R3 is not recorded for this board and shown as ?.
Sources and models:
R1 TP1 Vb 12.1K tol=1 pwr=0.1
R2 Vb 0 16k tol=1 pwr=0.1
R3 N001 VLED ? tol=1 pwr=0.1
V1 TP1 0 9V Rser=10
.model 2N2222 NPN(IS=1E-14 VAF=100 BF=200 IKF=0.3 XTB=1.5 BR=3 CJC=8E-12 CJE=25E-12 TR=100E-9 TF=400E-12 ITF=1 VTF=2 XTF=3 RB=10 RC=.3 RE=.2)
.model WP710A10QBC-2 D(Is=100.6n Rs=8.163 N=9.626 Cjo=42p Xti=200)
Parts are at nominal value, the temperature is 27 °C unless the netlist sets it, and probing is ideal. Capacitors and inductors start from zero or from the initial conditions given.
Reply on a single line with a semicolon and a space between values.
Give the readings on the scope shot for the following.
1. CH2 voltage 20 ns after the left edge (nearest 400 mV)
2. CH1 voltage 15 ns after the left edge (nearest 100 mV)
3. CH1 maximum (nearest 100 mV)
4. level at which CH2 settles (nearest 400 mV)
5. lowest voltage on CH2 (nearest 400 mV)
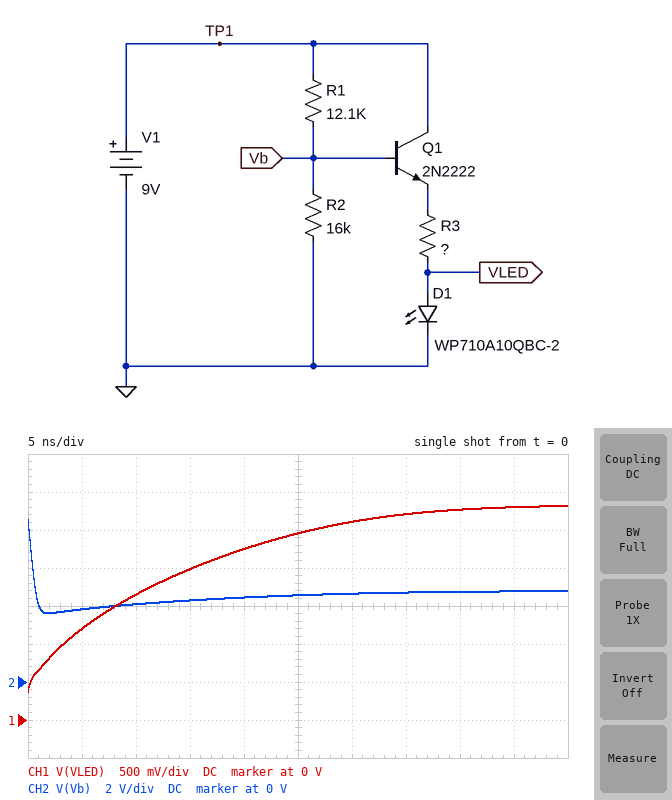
4.4 V; 2.0 V; 2.8 V; 4.8 V; 3.6 V
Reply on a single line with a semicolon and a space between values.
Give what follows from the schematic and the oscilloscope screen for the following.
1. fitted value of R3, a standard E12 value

180 Ω
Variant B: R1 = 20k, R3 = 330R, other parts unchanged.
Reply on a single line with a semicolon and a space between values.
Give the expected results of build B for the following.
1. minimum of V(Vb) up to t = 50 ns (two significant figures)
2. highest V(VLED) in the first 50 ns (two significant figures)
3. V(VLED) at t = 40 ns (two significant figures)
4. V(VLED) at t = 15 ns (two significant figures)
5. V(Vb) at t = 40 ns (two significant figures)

4.0 V; 2.4 V; 2.3 V; 1.6 V; 4.2 V
